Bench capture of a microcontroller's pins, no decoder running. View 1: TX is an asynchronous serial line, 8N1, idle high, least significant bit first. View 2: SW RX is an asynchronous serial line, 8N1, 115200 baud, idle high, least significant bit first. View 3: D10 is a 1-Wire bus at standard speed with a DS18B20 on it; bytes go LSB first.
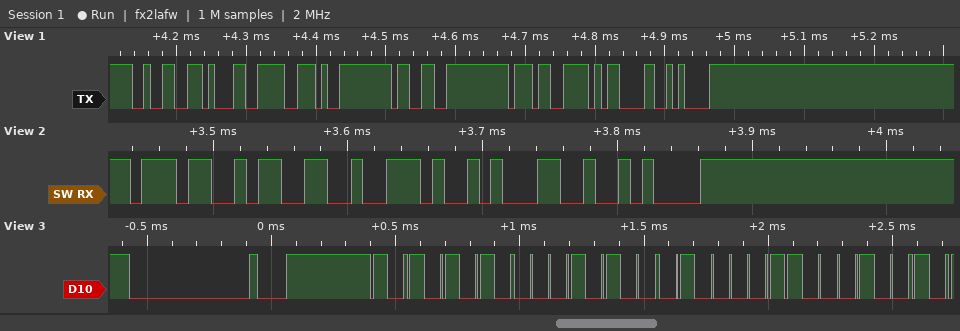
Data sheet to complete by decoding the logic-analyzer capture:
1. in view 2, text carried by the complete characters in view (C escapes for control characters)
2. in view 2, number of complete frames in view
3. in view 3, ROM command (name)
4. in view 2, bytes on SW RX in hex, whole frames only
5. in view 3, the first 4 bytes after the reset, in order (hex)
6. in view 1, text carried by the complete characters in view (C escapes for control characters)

"73.1\n"
5
Match ROM
0x37 0x33 0x2E 0x31 0x0A
55 28 C2 48
"21.37\r\n"
